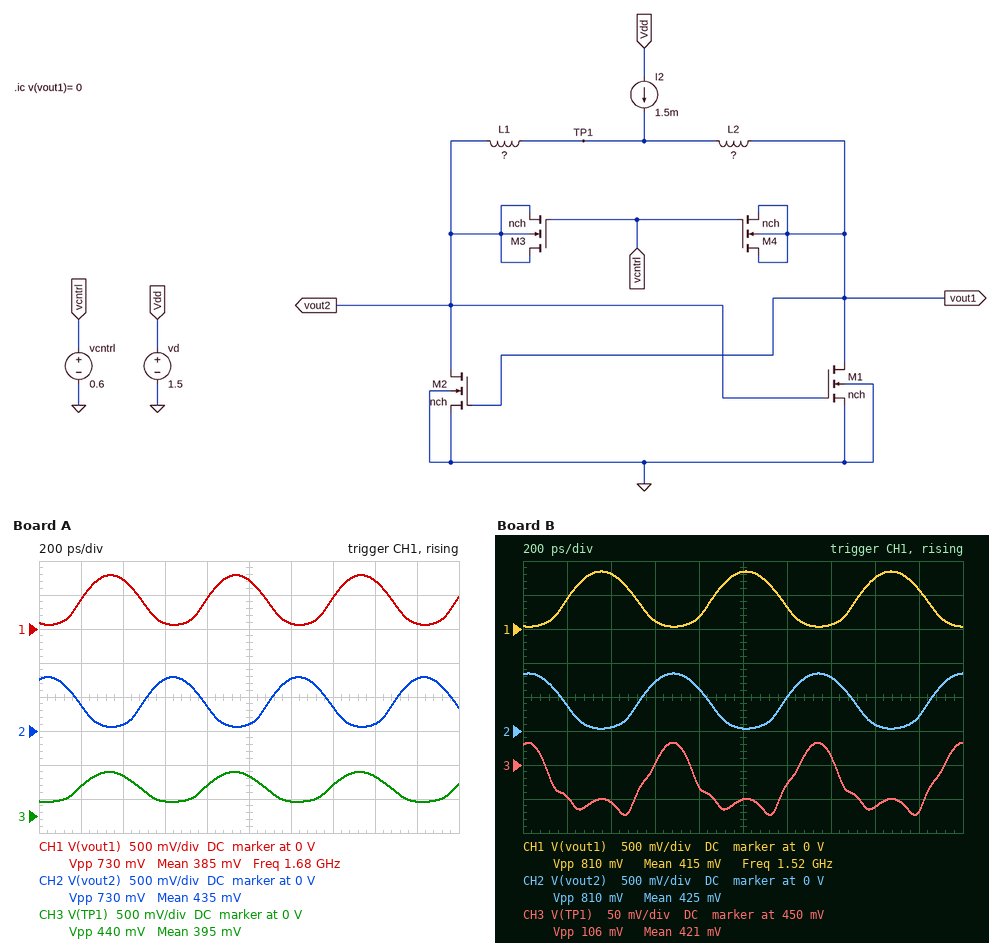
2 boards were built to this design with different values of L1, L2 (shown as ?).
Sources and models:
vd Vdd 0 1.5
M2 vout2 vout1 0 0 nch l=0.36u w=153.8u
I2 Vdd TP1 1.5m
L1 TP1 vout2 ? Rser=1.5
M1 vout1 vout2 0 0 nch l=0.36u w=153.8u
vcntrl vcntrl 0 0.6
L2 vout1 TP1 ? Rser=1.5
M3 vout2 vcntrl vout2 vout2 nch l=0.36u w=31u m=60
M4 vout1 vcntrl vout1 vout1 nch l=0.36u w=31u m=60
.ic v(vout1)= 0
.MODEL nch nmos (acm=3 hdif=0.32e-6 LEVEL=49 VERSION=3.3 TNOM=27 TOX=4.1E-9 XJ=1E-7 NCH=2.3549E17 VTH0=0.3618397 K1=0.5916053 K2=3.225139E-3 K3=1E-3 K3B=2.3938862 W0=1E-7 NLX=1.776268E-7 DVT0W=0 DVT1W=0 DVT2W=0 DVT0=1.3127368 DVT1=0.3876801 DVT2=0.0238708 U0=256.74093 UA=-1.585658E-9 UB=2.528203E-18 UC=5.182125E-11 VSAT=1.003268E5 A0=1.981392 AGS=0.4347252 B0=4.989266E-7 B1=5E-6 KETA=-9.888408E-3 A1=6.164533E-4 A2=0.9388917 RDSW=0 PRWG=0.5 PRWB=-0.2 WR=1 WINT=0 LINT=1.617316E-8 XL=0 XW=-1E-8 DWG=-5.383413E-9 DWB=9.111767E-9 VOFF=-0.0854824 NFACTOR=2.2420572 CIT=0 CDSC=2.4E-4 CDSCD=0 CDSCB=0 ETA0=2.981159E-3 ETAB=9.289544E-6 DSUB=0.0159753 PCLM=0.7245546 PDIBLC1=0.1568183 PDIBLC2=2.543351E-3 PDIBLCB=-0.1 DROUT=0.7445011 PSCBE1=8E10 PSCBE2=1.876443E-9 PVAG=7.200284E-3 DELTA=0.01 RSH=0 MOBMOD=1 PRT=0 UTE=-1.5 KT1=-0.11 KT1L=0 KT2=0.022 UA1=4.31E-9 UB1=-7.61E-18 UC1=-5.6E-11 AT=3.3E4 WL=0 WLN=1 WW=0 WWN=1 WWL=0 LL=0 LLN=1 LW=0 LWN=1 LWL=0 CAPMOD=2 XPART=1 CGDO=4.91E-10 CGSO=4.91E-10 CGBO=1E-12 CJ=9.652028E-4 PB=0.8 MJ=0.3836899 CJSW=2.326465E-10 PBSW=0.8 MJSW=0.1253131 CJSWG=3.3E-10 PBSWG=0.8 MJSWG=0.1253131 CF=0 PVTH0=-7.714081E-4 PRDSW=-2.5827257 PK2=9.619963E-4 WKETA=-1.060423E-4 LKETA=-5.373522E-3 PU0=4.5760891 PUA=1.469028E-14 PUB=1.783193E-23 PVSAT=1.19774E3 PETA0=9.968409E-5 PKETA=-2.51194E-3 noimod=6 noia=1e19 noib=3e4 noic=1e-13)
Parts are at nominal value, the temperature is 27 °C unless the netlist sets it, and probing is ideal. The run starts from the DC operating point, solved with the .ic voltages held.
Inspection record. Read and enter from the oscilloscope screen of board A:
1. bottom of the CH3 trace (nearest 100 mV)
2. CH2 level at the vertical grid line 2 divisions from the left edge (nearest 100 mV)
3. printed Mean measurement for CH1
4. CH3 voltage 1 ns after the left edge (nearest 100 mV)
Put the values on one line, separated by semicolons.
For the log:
200 mV; 100 mV; 385 mV; 600 mV
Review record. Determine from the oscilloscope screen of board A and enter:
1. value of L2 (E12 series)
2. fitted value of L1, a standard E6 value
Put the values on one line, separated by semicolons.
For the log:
820 pH; 3.3 nH
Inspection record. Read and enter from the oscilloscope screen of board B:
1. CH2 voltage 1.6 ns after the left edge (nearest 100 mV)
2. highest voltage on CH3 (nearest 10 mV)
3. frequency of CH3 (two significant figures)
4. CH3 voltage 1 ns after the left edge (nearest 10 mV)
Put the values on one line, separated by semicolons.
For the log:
100 mV; 480 mV; 1.5 GHz; 400 mV
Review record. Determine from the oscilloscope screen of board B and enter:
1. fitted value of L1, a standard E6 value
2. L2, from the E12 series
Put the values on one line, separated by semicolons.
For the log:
2.2 nH; 2.7 nH
